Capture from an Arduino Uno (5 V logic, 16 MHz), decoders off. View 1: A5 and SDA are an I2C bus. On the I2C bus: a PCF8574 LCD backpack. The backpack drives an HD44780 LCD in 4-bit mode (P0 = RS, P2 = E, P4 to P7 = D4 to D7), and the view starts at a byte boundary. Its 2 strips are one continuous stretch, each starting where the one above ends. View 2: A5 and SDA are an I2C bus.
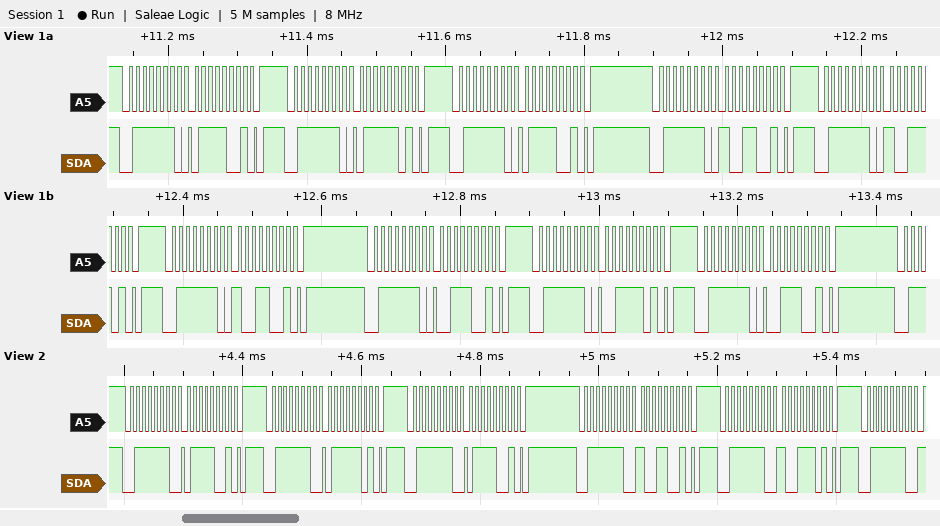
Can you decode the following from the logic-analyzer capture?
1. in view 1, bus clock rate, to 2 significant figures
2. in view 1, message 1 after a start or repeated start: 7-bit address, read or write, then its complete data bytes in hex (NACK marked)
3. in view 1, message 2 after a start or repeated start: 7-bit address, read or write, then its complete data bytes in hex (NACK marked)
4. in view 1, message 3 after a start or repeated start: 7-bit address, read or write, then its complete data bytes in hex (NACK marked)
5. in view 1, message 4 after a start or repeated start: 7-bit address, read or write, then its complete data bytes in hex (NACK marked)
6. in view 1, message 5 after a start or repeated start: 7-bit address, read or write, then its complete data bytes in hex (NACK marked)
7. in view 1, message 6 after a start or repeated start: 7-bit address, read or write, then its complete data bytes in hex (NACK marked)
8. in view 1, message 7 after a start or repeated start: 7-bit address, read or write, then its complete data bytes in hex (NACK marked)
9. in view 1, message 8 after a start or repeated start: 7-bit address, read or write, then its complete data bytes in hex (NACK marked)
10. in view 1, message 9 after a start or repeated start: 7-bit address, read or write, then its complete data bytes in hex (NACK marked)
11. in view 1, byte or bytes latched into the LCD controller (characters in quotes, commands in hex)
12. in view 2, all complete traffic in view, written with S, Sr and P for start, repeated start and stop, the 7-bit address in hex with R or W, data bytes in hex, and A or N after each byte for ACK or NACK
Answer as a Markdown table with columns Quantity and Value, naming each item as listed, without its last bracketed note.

| Quantity | Value |
|---|---|
| in view 1, bus clock rate, to 2 significant figures | 100 kHz |
| in view 1, message 1 after a start or repeated start: 7-bit address, read or write, then its complete data bytes in hex | 0x3F write: 79 |
| in view 1, message 2 after a start or repeated start: 7-bit address, read or write, then its complete data bytes in hex | 0x3F write: 7D |
| in view 1, message 3 after a start or repeated start: 7-bit address, read or write, then its complete data bytes in hex | 0x3F write: 79 |
| in view 1, message 4 after a start or repeated start: 7-bit address, read or write, then its complete data bytes in hex | 0x3F write: 99 |
| in view 1, message 5 after a start or repeated start: 7-bit address, read or write, then its complete data bytes in hex | 0x3F write: 9D |
| in view 1, message 6 after a start or repeated start: 7-bit address, read or write, then its complete data bytes in hex | 0x3F write: 99 |
| in view 1, message 7 after a start or repeated start: 7-bit address, read or write, then its complete data bytes in hex | 0x3F write: 39 |
| in view 1, message 8 after a start or repeated start: 7-bit address, read or write, then its complete data bytes in hex | 0x3F write: 3D |
| in view 1, message 9 after a start or repeated start: 7-bit address, read or write, then its complete data bytes in hex | 0x3F write: 39 |
| in view 1, byte or bytes latched into the LCD controller | 'y' |
| in view 2, all complete traffic in view, written with S, Sr and P for start, repeated start and stop, the 7-bit address in hex with R or W, data bytes in hex, and A or N after each byte for ACK or NACK | S 3FW A 79 A P S 3FW A 7D A P S 3FW A 79 A P S 3FW A 99 A P S 3FW A 9D A P S 3FW A |
